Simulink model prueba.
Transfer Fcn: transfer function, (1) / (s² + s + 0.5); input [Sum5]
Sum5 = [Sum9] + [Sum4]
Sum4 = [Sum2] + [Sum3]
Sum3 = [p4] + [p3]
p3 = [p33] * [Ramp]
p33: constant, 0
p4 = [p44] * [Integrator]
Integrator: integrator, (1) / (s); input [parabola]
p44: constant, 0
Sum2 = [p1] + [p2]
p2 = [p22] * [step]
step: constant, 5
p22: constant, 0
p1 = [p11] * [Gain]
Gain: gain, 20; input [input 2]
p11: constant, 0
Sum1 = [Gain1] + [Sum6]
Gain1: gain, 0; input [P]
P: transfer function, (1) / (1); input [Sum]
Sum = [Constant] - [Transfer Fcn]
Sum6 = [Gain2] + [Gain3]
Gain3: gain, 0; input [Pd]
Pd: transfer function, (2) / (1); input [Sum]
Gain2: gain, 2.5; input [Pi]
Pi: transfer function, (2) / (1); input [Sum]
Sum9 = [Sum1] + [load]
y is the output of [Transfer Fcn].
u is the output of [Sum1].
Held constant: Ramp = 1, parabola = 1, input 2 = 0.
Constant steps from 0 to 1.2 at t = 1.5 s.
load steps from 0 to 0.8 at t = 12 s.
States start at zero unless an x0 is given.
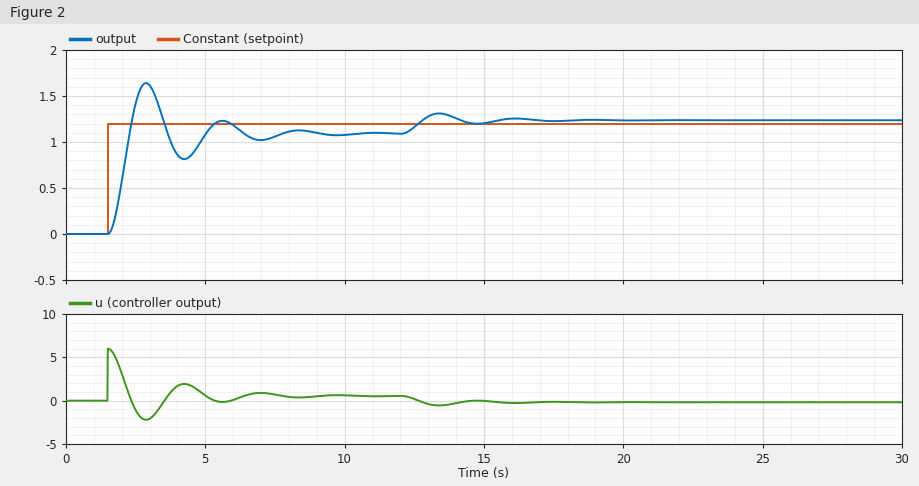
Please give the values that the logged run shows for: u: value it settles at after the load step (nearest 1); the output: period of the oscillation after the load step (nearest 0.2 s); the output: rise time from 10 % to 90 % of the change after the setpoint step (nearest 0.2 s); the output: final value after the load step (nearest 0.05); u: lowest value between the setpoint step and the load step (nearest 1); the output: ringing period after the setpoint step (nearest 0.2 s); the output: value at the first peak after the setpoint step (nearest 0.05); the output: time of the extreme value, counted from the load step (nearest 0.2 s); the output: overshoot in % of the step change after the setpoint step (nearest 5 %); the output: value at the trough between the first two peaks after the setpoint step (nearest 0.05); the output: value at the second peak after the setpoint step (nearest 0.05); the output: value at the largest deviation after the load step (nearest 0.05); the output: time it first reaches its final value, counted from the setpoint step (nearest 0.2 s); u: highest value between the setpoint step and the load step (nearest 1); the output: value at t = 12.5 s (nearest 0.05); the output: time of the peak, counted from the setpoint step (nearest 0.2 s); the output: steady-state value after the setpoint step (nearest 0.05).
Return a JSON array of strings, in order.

["0", "2.8 s", "0.6 s", "1.25", "-2", "2.8 s", "1.65", "1.4 s", "50 %", "0.80", "1.25", "1.30", "0.8 s", "6", "1.15", "1.4 s", "1.10"]
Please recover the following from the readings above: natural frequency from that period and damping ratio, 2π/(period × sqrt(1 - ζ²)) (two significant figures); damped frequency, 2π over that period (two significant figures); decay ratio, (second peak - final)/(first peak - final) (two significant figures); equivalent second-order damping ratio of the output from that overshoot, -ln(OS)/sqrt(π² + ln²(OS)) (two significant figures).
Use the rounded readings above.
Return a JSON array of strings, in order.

["2.3 rad/s", "2.2 rad/s", "0.27", "0.22"]
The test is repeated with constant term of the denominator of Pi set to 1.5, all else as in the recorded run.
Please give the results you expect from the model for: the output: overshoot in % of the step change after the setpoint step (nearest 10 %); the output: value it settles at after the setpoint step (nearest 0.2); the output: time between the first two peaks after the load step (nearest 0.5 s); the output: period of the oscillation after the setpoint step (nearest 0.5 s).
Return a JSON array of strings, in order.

["40 %", "1.0", "3.5 s", "3.5 s"]
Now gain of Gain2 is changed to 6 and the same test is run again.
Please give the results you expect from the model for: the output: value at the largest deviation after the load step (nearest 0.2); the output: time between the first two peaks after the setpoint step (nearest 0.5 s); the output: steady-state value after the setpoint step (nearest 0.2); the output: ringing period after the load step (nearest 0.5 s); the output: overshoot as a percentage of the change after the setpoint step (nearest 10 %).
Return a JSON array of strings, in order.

["1.2", "2.0 s", "1.2", "2.0 s", "60 %"]
